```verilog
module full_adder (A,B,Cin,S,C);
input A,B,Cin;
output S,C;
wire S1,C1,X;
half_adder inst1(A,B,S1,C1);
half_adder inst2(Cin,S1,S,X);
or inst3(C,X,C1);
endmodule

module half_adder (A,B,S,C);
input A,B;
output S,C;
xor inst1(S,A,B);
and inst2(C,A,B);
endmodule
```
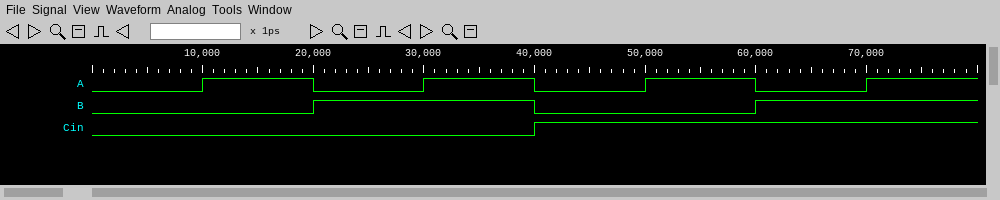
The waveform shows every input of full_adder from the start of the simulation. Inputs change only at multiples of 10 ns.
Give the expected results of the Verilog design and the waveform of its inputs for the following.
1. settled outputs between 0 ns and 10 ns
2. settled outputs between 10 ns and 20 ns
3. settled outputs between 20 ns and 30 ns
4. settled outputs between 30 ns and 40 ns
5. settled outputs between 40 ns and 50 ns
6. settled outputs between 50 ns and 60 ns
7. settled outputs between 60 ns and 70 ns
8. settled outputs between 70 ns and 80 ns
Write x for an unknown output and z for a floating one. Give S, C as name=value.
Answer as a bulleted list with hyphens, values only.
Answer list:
- S=0, C=0
- S=1, C=0
- S=1, C=0
- S=0, C=1
- S=1, C=0
- S=0, C=1
- S=0, C=1
- S=1, C=1
